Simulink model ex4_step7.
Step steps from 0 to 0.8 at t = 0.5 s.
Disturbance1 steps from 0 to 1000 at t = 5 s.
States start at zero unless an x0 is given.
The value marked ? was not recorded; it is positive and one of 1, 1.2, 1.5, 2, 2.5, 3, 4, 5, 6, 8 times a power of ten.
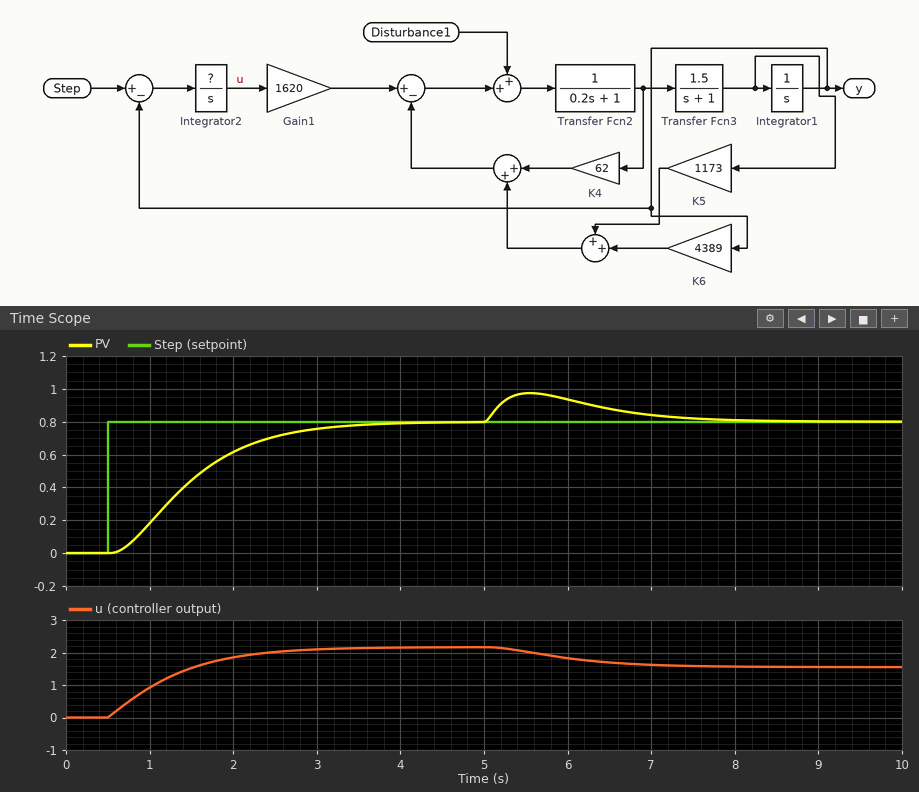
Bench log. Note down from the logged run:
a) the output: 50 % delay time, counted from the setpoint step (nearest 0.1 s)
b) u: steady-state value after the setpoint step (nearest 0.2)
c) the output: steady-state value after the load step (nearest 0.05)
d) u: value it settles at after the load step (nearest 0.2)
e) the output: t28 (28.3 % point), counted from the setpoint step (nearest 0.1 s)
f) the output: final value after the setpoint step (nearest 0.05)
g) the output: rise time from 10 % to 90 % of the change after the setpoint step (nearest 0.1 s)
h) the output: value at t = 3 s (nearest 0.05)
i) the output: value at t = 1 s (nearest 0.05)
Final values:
0.9 s
2.2
0.80
1.6
0.6 s
0.80
1.8 s
0.75
0.20
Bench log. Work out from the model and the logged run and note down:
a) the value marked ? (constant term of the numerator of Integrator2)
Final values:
2.5
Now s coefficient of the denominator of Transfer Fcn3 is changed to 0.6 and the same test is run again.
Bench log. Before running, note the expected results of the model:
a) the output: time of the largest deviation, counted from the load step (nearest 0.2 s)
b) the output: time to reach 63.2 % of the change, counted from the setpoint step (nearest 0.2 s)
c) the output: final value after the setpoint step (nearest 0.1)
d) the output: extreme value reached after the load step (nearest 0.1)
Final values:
0.6 s
1.2 s
0.8
1.0
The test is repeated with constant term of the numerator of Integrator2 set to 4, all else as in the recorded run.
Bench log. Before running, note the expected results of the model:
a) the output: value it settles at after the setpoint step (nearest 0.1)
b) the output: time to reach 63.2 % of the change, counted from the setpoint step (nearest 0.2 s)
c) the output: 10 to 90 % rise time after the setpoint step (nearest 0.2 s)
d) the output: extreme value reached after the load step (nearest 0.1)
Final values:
0.8
0.8 s
1.0 s
1.0
